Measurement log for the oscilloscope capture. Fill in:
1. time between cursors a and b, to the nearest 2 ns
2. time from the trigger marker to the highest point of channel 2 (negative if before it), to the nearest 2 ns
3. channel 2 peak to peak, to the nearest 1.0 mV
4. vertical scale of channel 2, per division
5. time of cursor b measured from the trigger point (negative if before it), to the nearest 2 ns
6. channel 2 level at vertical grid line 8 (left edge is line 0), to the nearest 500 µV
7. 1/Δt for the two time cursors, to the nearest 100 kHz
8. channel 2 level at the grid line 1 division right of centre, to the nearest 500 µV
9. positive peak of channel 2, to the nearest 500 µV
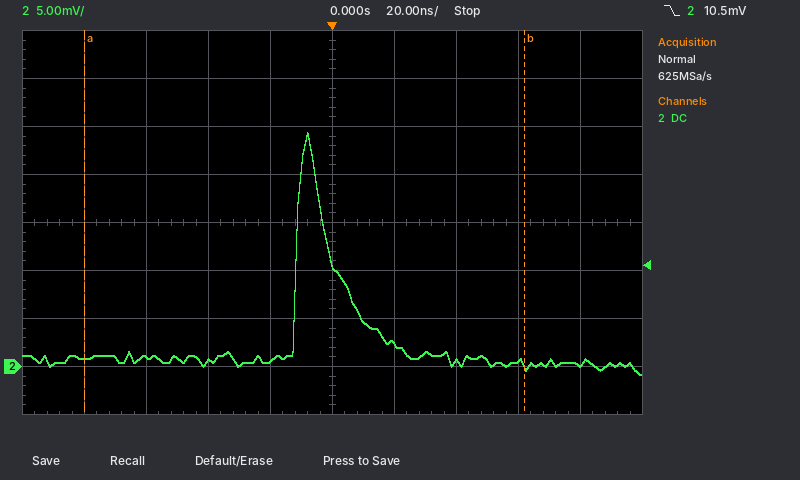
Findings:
142 ns
-8 ns
25.0 mV
5 mV
+62 ns
500 µV
7.0 MHz
2.5 mV
24.5 mV
